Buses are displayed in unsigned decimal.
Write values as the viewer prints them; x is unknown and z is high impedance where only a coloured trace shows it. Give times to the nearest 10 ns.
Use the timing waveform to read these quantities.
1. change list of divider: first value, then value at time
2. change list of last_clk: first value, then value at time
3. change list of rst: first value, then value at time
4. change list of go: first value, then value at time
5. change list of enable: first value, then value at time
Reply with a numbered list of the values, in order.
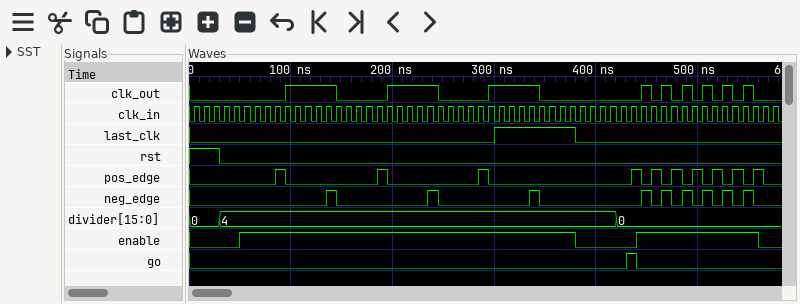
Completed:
1. 0, 4 at 30 ns, 0 at 420 ns
2. 0, 1 at 300 ns, 0 at 380 ns
3. 1, 0 at 30 ns
4. 0, 1 at 430 ns, 0 at 440 ns
5. 0, 1 at 50 ns, 0 at 380 ns, 1 at 440 ns, 0 at 560 ns
